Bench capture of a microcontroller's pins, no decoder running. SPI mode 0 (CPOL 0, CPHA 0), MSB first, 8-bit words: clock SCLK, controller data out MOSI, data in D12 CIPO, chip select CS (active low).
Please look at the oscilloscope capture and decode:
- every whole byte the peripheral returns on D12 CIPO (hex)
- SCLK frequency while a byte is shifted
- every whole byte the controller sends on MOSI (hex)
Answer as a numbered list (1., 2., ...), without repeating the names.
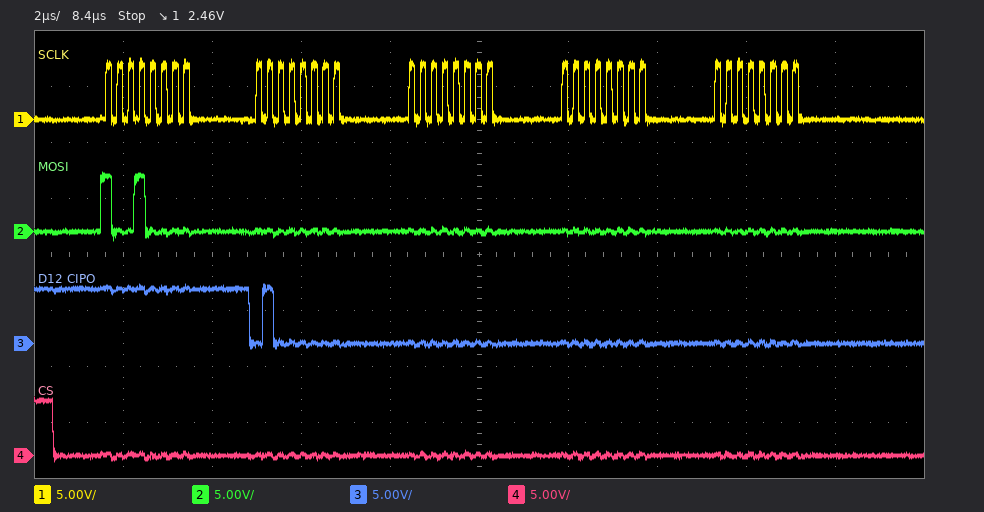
1. FF 40 00 00 00
2. 4 MHz
3. 90 00 00 00 00
